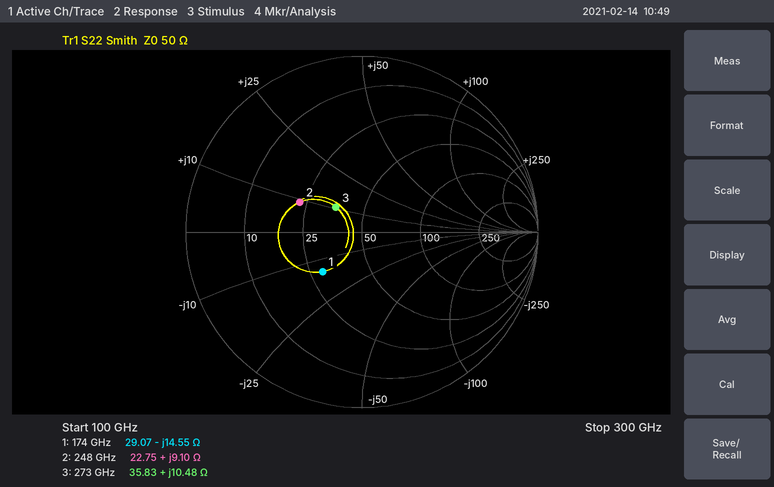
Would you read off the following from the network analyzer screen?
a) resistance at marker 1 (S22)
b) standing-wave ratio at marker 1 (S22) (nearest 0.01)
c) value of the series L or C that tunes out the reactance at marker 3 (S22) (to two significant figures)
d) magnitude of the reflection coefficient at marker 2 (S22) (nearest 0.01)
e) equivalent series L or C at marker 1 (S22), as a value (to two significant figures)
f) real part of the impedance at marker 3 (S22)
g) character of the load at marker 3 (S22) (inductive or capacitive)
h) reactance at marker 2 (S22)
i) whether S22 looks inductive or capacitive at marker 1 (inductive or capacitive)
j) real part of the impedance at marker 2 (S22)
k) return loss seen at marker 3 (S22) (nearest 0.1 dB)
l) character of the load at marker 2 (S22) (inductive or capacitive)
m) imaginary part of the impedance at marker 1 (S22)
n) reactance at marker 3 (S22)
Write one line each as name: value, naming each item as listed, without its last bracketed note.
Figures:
resistance at marker 1: 29.07 Ω
standing-wave ratio at marker 1 (S22): 1.93
value of the series L or C that tunes out the reactance at marker 3 (S22): 56 fF
magnitude of the reflection coefficient at marker 2 (S22): 0.39
equivalent series L or C at marker 1 (S22), as a value: 63 fF
real part of the impedance at marker 3: 35.83 Ω
character of the load at marker 3 (S22): inductive
reactance at marker 2: +9.10 Ω
whether S22 looks inductive or capacitive at marker 1: capacitive
real part of the impedance at marker 2: 22.75 Ω
return loss seen at marker 3 (S22): 13.8 dB
character of the load at marker 2 (S22): inductive
imaginary part of the impedance at marker 1: -14.55 Ω
reactance at marker 3: +10.48 Ω
